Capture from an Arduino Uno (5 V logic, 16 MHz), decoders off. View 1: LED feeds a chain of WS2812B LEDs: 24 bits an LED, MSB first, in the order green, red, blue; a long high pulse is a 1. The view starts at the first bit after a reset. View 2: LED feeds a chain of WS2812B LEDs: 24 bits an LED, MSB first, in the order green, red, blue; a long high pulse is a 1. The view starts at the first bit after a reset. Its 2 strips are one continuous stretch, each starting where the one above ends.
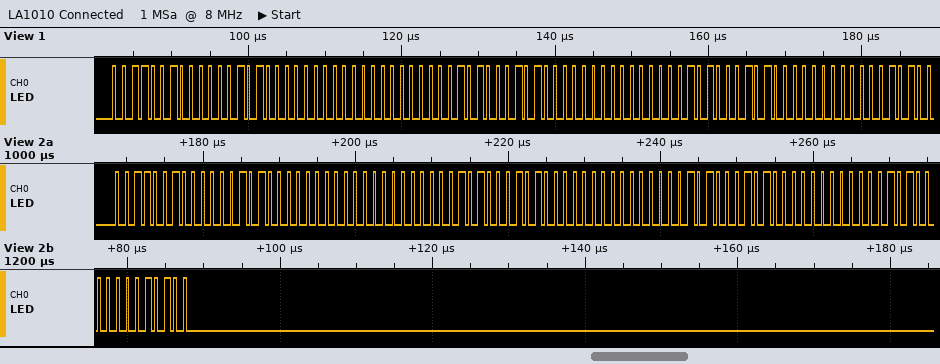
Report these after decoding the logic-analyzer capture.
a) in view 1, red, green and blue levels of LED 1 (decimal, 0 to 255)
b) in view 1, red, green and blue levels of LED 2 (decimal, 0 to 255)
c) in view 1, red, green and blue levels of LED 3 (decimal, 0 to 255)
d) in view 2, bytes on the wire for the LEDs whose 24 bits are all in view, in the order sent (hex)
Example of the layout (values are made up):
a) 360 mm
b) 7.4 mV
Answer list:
a) 5, 50, 0
b) 10, 0, 40
c) 10, 0, 40
d) 32 05 00 00 0A 28 00 0A 28 00 50 14
